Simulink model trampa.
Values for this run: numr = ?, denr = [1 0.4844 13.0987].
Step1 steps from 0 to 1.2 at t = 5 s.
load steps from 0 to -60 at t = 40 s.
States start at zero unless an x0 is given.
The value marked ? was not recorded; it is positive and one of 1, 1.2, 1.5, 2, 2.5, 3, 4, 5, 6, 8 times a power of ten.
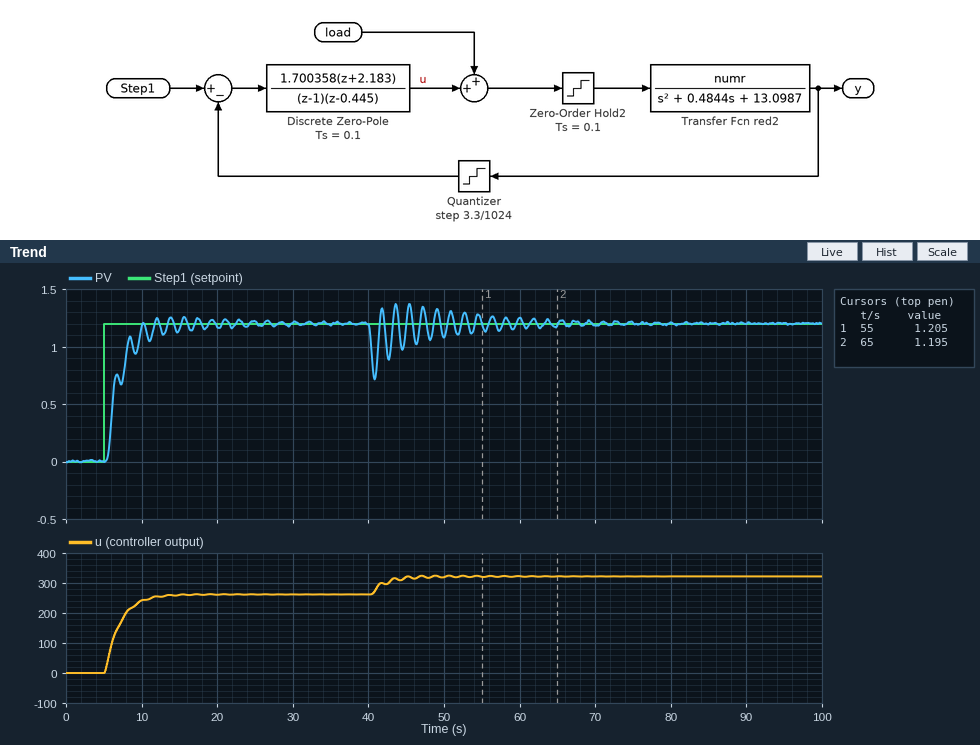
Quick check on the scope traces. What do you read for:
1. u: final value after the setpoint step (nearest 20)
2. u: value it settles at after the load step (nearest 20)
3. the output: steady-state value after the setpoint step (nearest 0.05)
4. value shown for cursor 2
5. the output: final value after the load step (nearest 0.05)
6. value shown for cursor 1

260
320
1.20
1.195
1.20
1.205
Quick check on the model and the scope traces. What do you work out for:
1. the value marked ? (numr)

0.06
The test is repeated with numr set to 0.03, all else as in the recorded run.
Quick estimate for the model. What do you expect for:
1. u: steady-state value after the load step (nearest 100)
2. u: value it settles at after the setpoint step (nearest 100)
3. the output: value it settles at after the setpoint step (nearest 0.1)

600
500
1.2
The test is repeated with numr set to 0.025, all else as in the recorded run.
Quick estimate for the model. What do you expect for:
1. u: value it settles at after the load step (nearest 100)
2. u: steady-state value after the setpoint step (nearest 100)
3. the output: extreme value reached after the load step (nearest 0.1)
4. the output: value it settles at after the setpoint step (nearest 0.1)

700
600
1.0
1.2
